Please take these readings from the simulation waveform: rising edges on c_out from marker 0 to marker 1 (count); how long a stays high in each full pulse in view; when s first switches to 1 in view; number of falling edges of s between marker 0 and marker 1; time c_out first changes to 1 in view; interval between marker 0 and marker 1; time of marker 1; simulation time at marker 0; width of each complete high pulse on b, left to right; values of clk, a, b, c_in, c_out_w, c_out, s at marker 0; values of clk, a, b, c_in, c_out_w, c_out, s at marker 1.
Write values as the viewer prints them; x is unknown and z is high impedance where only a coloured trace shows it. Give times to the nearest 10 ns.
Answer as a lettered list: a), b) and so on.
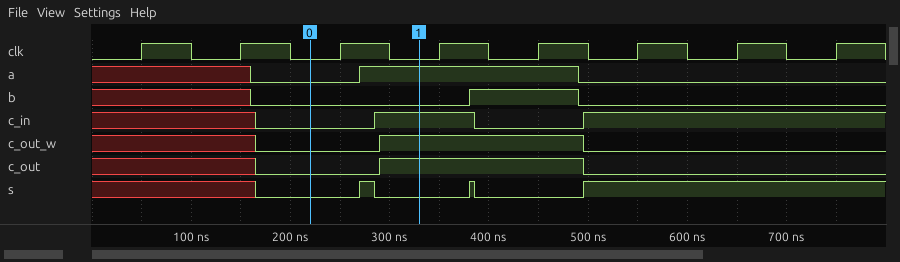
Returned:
a) 1
b) 220 ns
c) 270 ns
d) 1
e) 290 ns
f) 110 ns
g) 330 ns
h) 220 ns
i) 110 ns
j) clk=0, a=0, b=0, c_in=0, c_out_w=0, c_out=0, s=0
k) clk=0, a=1, b=0, c_in=1, c_out_w=1, c_out=1, s=0
